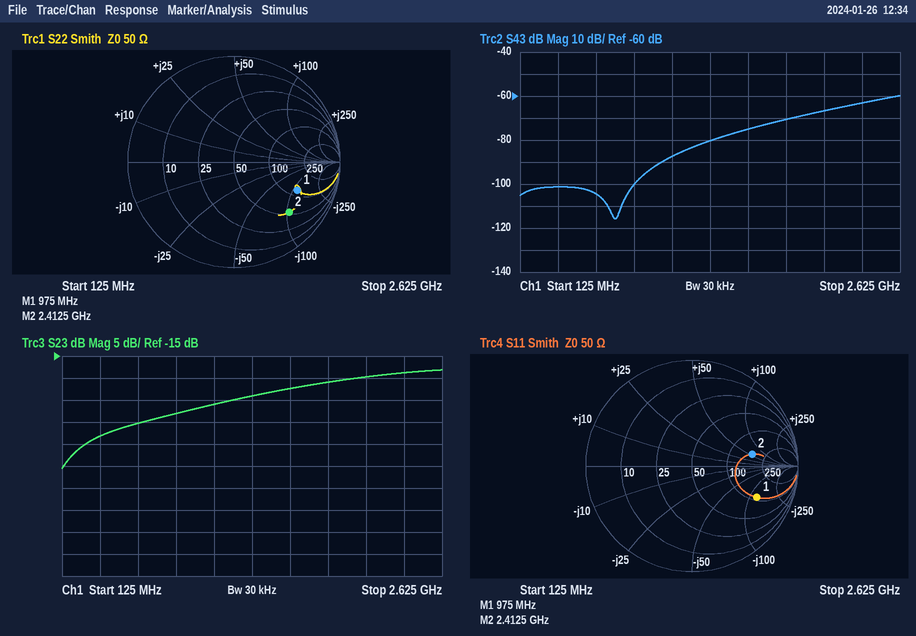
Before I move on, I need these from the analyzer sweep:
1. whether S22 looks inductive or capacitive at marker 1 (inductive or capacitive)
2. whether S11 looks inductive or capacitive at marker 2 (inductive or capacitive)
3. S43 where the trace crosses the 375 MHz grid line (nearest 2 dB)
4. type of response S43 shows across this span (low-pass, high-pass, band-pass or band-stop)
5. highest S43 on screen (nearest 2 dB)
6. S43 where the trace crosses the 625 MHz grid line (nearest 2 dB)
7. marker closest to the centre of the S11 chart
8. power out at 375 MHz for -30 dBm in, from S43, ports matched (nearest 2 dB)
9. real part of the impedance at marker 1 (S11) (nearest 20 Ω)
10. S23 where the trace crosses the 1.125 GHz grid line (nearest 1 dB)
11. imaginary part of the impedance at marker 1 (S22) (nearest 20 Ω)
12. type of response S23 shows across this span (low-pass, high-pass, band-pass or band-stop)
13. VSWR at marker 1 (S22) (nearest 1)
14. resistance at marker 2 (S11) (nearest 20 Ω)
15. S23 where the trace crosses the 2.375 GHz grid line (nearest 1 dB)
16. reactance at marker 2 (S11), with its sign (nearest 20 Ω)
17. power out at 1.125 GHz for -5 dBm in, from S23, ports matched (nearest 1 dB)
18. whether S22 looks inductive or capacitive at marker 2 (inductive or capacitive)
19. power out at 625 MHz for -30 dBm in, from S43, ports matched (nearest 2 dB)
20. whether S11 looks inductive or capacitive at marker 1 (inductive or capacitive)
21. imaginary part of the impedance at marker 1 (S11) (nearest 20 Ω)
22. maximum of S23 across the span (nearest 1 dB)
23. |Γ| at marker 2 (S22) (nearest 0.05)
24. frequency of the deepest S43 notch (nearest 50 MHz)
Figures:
capacitive
inductive
-102 dB
high-pass
-60 dB
-104 dB
marker 2
-132 dBm
120 Ω
-26 dB
-120 Ω
high-pass
5
160 Ω
-19 dB
+60 Ω
-31 dBm
capacitive
-134 dBm
capacitive
-120 Ω
-18 dB
0.70
750 MHz
